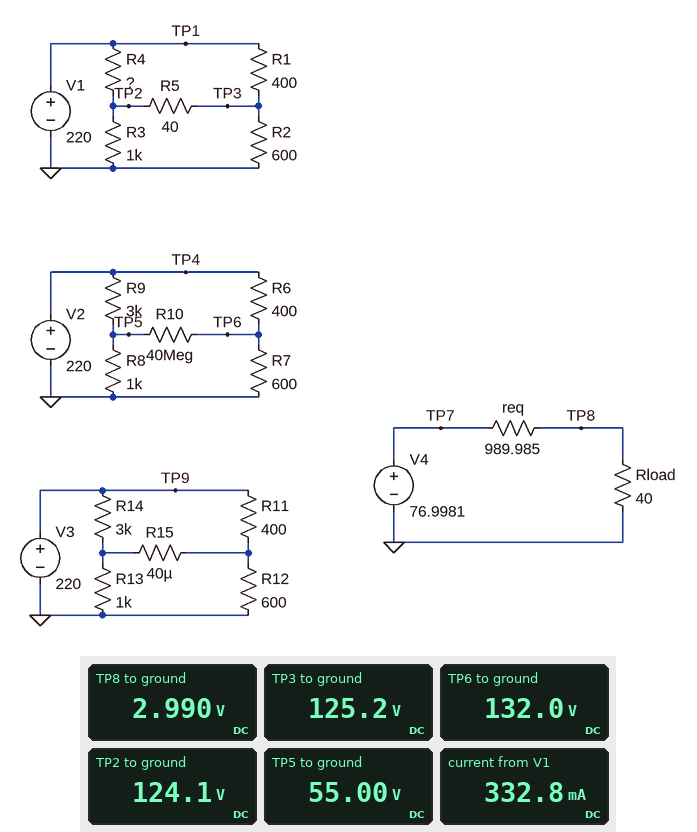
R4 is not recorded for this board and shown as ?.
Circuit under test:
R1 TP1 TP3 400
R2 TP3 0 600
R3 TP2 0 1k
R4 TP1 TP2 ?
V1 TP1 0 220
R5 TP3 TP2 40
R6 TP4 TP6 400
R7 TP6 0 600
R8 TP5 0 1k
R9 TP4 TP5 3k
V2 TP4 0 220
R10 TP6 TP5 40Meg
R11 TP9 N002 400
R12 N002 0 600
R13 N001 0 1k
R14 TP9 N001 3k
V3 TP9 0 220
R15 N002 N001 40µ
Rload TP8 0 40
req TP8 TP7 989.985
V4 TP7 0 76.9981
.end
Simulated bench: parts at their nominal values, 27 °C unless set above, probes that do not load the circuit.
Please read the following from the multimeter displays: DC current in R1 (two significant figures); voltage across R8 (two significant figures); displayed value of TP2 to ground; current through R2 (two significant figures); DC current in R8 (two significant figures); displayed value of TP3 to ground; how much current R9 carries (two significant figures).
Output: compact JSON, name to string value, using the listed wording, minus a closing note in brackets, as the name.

{"DC current in R1": "240 mA", "voltage across R8": "55 V", "displayed value of TP2 to ground": "124.1 V", "current through R2": "210 mA", "DC current in R8": "55 mA", "displayed value of TP3 to ground": "125.2 V", "how much current R9 carries": "55 mA"}
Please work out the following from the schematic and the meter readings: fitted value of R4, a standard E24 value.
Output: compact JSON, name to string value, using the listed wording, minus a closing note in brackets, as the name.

{"fitted value of R4, a standard E24 value": "1 kΩ"}
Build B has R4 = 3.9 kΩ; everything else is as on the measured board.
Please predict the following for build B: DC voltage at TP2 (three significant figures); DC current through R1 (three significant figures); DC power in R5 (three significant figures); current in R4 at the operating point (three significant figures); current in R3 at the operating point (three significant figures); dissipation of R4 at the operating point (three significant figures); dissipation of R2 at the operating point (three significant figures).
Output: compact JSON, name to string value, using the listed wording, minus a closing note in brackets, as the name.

{"DC voltage at TP2": "109 V", "DC current through R1": "269 mA", "DC power in R5": "262 mW", "current in R4 at the operating point": "28.4 mA", "current in R3 at the operating point": "109 mA", "dissipation of R4 at the operating point": "3.14 W", "dissipation of R2 at the operating point": "21.1 W"}
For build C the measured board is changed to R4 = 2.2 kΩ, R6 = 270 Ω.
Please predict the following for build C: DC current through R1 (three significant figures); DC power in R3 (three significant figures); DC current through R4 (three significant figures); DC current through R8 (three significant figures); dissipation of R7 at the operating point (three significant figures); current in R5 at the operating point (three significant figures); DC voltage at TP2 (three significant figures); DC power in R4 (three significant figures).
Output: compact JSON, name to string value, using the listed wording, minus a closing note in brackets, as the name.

{"DC current through R1": "259 mA", "DC power in R3": "12.9 W", "DC current through R4": "48.3 mA", "DC current through R8": "55.0 mA", "dissipation of R7 at the operating point": "38.4 W", "current in R5 at the operating point": "65.4 mA", "DC voltage at TP2": "114 V", "DC power in R4": "5.14 W"}
